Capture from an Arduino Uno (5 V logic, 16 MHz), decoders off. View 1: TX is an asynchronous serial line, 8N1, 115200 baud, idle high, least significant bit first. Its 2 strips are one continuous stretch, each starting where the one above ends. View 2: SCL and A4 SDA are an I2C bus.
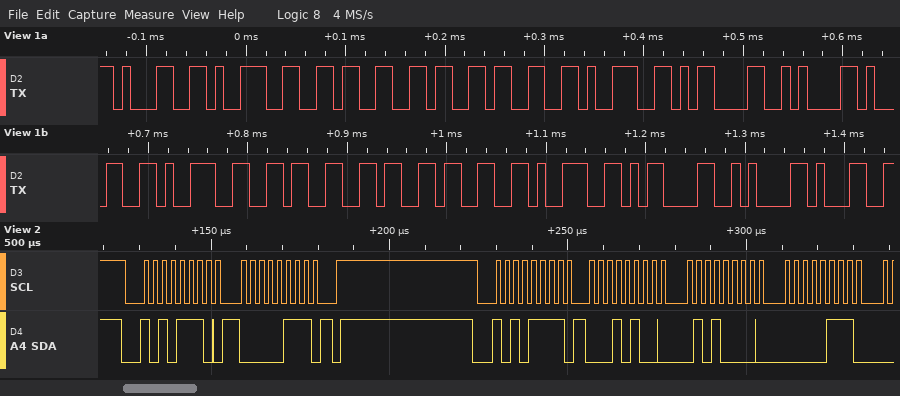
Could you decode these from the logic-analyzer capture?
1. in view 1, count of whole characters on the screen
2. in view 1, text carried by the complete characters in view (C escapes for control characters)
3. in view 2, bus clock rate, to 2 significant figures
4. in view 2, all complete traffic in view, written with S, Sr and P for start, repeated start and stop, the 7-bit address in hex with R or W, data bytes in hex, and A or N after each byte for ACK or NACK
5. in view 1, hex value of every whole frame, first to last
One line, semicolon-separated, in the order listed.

17; "196639\r\n196639\r\n1"; 400 kHz; S 57W A 07 A P S 57R A 14 A 50 A 07 A; 31 39 36 36 33 39 0D 0A 31 39 36 36 33 39 0D 0A 31
